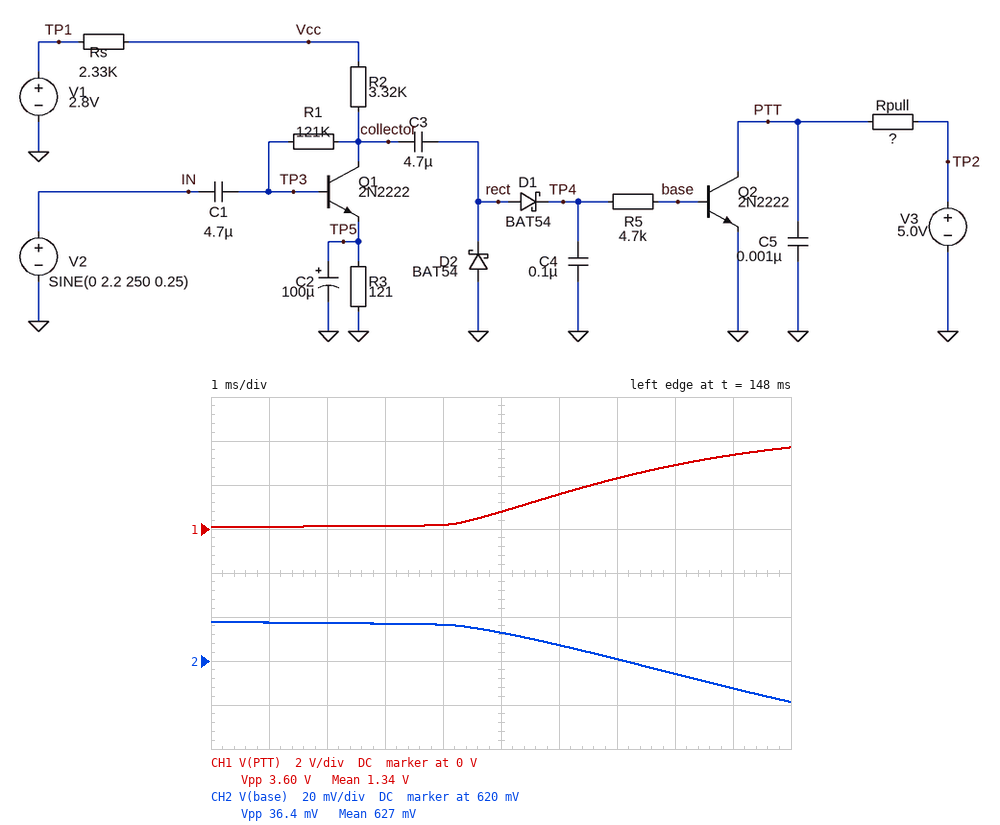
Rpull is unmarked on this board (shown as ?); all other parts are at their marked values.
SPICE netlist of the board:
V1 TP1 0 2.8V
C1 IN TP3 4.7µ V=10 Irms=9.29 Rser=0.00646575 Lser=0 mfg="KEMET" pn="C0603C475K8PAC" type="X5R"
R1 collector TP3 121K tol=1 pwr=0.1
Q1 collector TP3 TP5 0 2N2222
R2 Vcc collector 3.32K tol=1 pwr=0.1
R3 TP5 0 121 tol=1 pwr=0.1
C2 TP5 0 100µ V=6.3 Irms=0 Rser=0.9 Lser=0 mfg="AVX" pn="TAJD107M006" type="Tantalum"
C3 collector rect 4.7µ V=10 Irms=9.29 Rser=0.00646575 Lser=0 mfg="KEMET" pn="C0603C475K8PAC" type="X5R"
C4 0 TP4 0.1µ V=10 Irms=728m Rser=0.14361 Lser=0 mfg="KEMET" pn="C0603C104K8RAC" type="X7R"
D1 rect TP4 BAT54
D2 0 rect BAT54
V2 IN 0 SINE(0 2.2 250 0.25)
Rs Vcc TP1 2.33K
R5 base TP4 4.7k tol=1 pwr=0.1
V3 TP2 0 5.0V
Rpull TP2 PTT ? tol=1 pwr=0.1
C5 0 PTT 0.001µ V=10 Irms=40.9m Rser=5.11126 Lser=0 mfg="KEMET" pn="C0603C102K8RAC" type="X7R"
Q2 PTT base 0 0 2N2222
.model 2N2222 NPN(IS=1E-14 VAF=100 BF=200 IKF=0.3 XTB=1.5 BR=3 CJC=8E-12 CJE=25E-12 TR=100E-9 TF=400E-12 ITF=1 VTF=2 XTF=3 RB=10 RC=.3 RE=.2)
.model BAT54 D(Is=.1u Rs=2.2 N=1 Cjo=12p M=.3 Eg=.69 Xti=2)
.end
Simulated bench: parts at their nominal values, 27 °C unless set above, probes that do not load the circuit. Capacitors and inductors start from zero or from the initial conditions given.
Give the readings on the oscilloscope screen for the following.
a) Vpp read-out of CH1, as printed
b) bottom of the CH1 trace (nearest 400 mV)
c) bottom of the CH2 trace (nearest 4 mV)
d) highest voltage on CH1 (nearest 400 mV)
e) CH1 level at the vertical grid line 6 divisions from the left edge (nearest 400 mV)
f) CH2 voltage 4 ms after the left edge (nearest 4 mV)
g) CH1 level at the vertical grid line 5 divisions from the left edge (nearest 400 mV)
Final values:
3.60 V
0 V
600 mV
3.6 V
1.6 V
636 mV
800 mV
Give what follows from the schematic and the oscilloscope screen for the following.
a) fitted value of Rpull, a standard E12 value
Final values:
10 kΩ
